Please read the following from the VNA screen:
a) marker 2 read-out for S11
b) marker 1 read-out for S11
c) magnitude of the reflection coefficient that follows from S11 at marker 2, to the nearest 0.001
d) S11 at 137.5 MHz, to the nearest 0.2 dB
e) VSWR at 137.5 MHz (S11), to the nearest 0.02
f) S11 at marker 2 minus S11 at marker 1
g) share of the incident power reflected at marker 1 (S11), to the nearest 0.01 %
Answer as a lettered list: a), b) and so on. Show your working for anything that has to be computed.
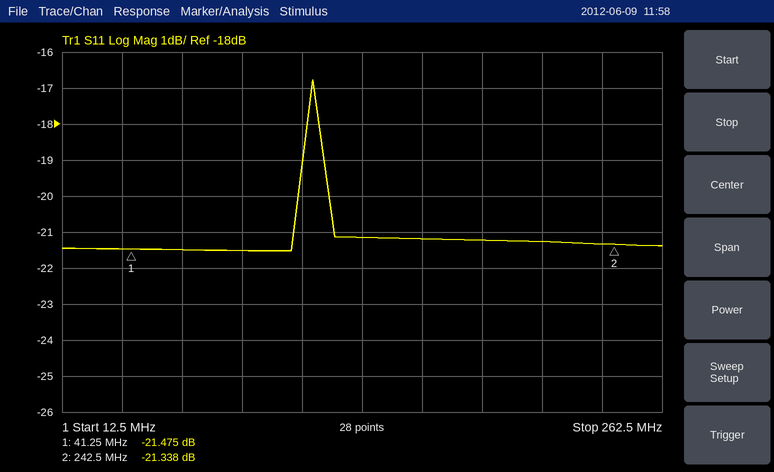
a) -21.338 dB
b) -21.475 dB
c) 10^(-21.338/20) ≈ 0.086
d) -21.2 dB
e) |Γ| = 10^(-21.2/20) = 0.0871; VSWR = (1 + 0.0871)/(1 − 0.0871) ≈ 1.19, so 1.20 to the nearest 0.02
f) -21.338 − (-21.475) = 0.137 dB
g) 10^(-21.475/10) ≈ 0.71 %
